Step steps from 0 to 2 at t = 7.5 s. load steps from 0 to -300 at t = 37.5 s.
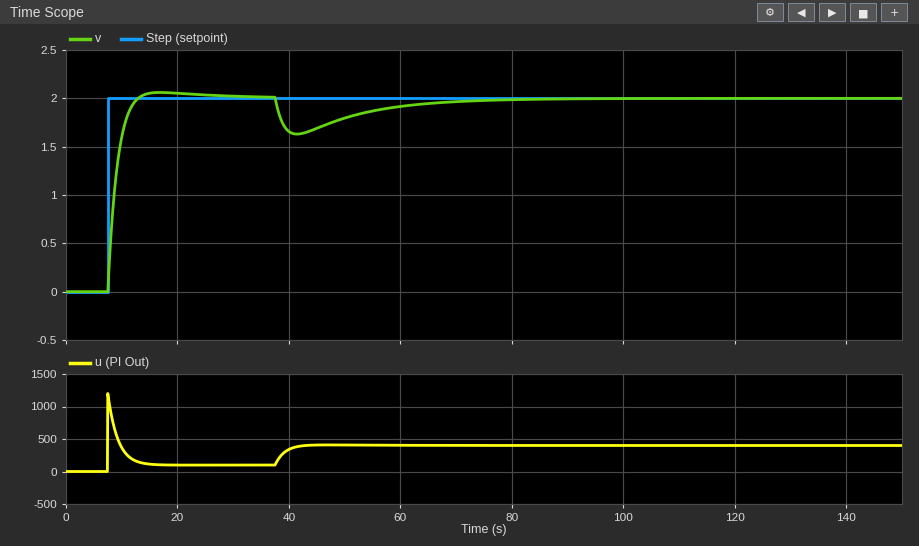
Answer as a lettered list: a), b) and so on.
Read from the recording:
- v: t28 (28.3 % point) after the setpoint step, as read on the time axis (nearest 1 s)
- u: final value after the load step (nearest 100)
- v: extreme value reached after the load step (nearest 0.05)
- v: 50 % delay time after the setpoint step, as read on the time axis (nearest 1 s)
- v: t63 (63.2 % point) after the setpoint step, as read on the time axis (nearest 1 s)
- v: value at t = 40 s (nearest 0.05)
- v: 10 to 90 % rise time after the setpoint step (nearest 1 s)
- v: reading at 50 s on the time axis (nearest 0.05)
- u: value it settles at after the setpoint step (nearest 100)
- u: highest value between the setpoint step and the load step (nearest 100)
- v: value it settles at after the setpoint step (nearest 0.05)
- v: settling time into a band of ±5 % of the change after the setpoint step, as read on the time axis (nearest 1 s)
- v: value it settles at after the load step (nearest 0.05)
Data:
a) 8 s
b) 400
c) 1.65
d) 9 s
e) 9 s
f) 1.65
g) 3 s
h) 1.80
i) 100
j) 1200
k) 2.00
l) 12 s
m) 2.00
